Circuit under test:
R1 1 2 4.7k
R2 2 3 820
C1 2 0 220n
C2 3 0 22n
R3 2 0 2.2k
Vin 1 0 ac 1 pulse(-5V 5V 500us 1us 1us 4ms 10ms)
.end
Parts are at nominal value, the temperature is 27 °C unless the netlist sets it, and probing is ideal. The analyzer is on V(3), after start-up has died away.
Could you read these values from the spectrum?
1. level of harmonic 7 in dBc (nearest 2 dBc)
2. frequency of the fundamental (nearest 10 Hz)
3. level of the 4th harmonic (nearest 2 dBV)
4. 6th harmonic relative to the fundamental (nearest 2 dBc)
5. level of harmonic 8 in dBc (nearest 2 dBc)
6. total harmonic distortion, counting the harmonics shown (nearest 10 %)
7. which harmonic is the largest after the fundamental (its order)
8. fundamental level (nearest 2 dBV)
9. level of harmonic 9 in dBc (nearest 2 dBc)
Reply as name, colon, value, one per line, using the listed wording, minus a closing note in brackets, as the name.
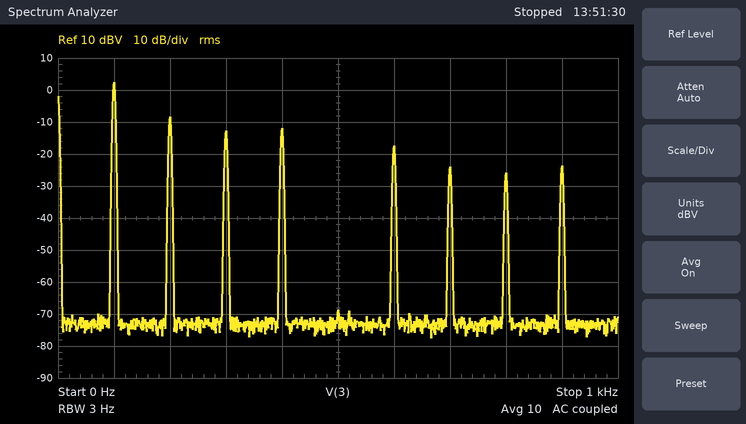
level of harmonic 7 in dBc: -26 dBc
frequency of the fundamental: 100 Hz
level of the 4th harmonic: -12 dBV
6th harmonic relative to the fundamental: -20 dBc
level of harmonic 8 in dBc: -28 dBc
total harmonic distortion, counting the harmonics shown: 40 %
which harmonic is the largest after the fundamental: 2
fundamental level: 2 dBV
level of harmonic 9 in dBc: -26 dBc
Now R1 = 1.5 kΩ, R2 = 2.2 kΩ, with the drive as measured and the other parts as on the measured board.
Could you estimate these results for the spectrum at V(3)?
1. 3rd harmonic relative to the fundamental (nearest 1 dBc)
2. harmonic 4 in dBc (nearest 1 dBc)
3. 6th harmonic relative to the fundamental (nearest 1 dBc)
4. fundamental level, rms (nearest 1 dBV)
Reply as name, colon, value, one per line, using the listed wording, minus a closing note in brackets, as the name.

3rd harmonic relative to the fundamental: -14 dBc
harmonic 4 in dBc: -13 dBc
6th harmonic relative to the fundamental: -18 dBc
fundamental level, rms: 8 dBV
